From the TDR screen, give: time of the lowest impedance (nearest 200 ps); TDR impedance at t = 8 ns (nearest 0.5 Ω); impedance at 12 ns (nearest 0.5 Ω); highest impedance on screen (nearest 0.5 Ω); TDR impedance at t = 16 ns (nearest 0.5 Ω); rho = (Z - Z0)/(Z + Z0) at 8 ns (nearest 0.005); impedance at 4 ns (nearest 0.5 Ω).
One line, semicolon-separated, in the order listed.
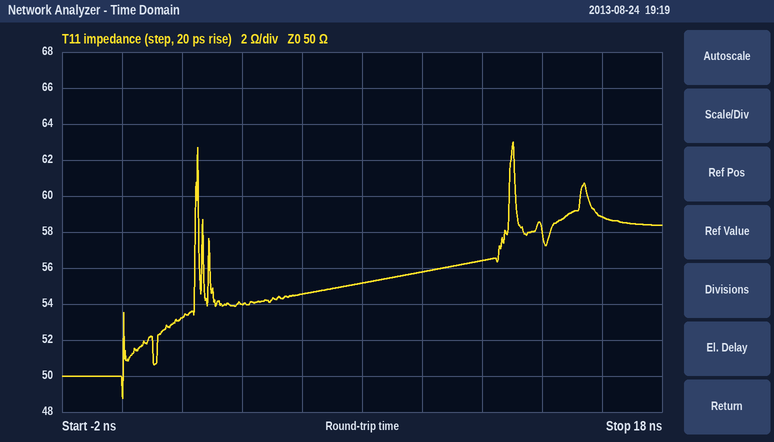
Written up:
0.0 ns; 55.0 Ω; 56.5 Ω; 63.0 Ω; 59.0 Ω; +0.050; 54.0 Ω
